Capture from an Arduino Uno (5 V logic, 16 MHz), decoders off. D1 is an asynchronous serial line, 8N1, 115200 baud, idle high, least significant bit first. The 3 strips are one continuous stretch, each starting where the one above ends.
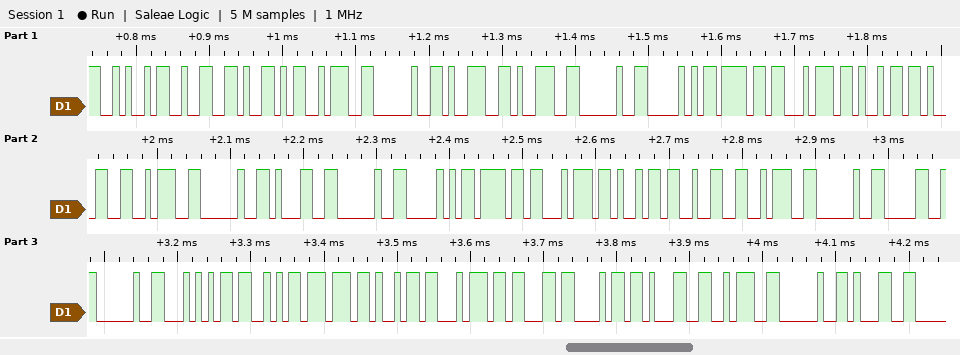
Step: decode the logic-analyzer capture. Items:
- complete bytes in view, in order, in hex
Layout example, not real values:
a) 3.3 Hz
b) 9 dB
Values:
a) 4A 32 59 3A 20 39 39 20 50 6F 74 69 31 3A 20 31 20 50 6F 74 69 32 3A 20 30 20 54 53 77 69 74 63 68 31 3A 20 31
